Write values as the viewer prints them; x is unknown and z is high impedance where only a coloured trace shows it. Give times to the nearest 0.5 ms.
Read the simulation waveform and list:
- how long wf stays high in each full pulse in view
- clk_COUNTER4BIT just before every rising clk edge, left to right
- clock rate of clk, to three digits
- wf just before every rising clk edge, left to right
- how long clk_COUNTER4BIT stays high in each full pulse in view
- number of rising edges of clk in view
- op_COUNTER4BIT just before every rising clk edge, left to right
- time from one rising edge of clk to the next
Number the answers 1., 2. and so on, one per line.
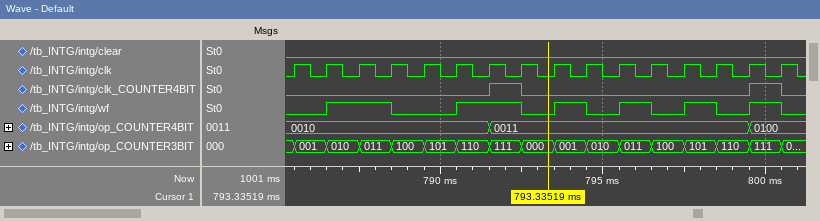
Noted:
1. 2 ms, 2 ms, 1 ms, 1 ms, 1 ms, 1 ms
2. 0 0 0 0 0 0 0 1 0 0 0 0 0 0 0 1
3. 1.00 kHz
4. 0 0 1 1 0 0 1 1 0 1 0 1 0 1 0 1
5. 1 ms, 1 ms
6. 16
7. 0010, 0010, 0010, 0010, 0010, 0010, 0010, 0011, 0011, 0011, 0011, 0011, 0011, 0011, 0011, 0100
8. 1 ms
